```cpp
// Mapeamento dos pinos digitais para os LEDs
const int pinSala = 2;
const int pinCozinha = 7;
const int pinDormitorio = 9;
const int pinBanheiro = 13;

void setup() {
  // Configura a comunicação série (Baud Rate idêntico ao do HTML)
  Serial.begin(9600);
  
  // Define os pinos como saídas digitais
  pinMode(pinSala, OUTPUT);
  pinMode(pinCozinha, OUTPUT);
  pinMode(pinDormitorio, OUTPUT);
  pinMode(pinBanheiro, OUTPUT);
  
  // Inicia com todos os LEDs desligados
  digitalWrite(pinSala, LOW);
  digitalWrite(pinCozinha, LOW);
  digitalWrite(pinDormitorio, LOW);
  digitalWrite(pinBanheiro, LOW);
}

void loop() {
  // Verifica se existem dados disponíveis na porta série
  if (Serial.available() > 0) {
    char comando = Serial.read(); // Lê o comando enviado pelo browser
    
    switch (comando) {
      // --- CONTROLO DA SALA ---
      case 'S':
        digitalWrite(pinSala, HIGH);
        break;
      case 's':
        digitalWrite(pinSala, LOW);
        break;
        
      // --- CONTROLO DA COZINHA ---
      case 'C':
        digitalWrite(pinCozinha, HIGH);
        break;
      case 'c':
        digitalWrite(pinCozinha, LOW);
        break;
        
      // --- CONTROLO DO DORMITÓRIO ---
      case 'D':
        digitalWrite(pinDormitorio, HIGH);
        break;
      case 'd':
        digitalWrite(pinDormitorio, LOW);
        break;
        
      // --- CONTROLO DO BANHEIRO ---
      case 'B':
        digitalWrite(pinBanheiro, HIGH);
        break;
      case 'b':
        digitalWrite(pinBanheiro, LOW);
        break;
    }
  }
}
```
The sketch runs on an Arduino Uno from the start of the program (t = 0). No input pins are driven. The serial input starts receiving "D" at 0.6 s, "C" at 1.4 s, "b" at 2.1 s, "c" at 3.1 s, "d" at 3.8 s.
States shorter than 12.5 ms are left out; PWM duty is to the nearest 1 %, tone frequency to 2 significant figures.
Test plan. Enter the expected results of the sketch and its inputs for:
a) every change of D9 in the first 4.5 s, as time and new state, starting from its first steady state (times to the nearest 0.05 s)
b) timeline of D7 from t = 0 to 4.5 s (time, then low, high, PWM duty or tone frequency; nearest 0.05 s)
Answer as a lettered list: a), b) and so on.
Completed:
a) 0 s low; 0.6 s high; 3.8 s low
b) 0 s low; 1.4 s high; 3.1 s low
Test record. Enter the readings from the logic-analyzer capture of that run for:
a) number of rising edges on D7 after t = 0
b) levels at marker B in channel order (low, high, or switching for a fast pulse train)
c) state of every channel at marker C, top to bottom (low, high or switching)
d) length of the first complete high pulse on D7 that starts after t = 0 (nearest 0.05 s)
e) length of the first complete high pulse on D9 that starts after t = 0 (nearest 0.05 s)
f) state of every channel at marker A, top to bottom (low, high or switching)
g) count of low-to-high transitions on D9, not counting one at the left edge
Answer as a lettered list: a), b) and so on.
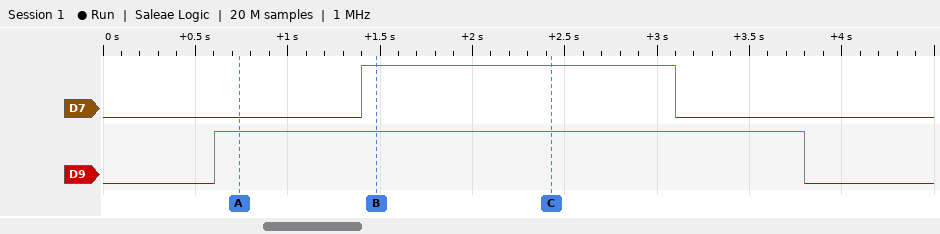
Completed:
a) 1
b) D7 high, D9 high
c) D7 high, D9 high
d) 1.70 s
e) 3.20 s
f) D7 low, D9 high
g) 1
